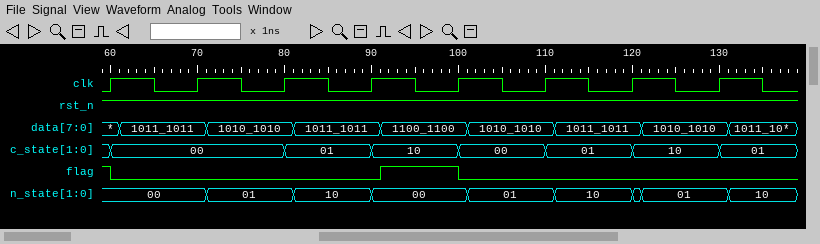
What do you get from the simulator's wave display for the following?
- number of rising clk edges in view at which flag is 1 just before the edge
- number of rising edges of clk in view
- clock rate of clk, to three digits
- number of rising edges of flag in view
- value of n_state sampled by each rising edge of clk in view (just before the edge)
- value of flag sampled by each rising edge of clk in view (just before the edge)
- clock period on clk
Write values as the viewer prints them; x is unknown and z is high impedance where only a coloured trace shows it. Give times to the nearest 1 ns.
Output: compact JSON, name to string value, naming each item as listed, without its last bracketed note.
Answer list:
{"number of rising clk edges in view at which flag is 1 just before the edge": "2", "number of rising edges of clk in view": "8", "clock rate of clk, to three digits": "100 MHz", "number of rising edges of flag in view": "1", "value of n_state sampled by each rising edge of clk in view": "00, 00, 01, 10, 00, 01, 10, 01", "value of flag sampled by each rising edge of clk in view": "1 0 0 0 1 0 0 0", "clock period on clk": "10 ns"}
